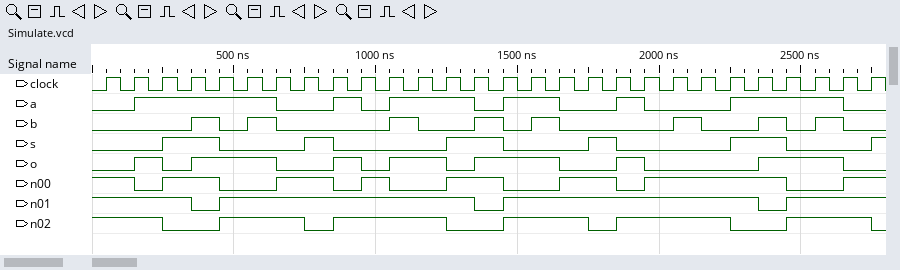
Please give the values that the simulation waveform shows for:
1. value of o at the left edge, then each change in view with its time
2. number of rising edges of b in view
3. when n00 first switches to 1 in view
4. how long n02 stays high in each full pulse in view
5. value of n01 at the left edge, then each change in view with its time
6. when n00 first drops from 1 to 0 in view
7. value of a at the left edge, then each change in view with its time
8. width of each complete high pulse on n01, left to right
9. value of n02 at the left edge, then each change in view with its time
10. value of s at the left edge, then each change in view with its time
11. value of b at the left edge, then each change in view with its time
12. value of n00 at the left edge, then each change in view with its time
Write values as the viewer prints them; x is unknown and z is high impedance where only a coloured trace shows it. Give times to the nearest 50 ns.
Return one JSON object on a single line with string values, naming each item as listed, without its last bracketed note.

{"value of o at the left edge, then each change in view with its time": "0, 1 at 150 ns, 0 at 250 ns, 1 at 350 ns, 0 at 650 ns, 1 at 850 ns, 0 at 950 ns, 1 at 1050 ns, 0 at 1250 ns, 1 at 1350 ns, 0 at 1650 ns, 1 at 1850 ns, 0 at 1950 ns, 1 at 2350 ns, 0 at 2650 ns", "number of rising edges of b in view": "8", "when n00 first switches to 1 in view": "250 ns", "how long n02 stays high in each full pulse in view": "300 ns, 400 ns, 300 ns, 400 ns, 300 ns", "value of n01 at the left edge, then each change in view with its time": "1, 0 at 350 ns, 1 at 450 ns, 0 at 1350 ns, 1 at 1450 ns, 0 at 2350 ns, 1 at 2450 ns", "when n00 first drops from 1 to 0 in view": "150 ns", "value of a at the left edge, then each change in view with its time": "0, 1 at 150 ns, 0 at 650 ns, 1 at 850 ns, 0 at 950 ns, 1 at 1050 ns, 0 at 1350 ns, 1 at 1450 ns, 0 at 1650 ns, 1 at 1850 ns, 0 at 1950 ns, 1 at 2250 ns, 0 at 2650 ns", "width of each complete high pulse on n01, left to right": "900 ns, 900 ns", "value of n02 at the left edge, then each change in view with its time": "1, 0 at 250 ns, 1 at 450 ns, 0 at 750 ns, 1 at 850 ns, 0 at 1250 ns, 1 at 1450 ns, 0 at 1750 ns, 1 at 1850 ns, 0 at 2250 ns, 1 at 2450 ns, 0 at 2750 ns", "value of s at the left edge, then each change in view with its time": "0, 1 at 250 ns, 0 at 450 ns, 1 at 750 ns, 0 at 850 ns, 1 at 1250 ns, 0 at 1450 ns, 1 at 1750 ns, 0 at 1850 ns, 1 at 2250 ns, 0 at 2450 ns, 1 at 2750 ns", "value of b at the left edge, then each change in view with its time": "0, 1 at 350 ns, 0 at 450 ns, 1 at 550 ns, 0 at 650 ns, 1 at 1050 ns, 0 at 1150 ns, 1 at 1350 ns, 0 at 1450 ns, 1 at 1550 ns, 0 at 1650 ns, 1 at 2050 ns, 0 at 2150 ns, 1 at 2350 ns, 0 at 2450 ns, 1 at 2550 ns, 0 at 2650 ns", "value of n00 at the left edge, then each change in view with its time": "1, 0 at 150 ns, 1 at 250 ns, 0 at 450 ns, 1 at 650 ns, 0 at 850 ns, 1 at 950 ns, 0 at 1050 ns, 1 at 1250 ns, 0 at 1450 ns, 1 at 1650 ns, 0 at 1850 ns, 1 at 1950 ns, 0 at 2450 ns, 1 at 2650 ns"}
